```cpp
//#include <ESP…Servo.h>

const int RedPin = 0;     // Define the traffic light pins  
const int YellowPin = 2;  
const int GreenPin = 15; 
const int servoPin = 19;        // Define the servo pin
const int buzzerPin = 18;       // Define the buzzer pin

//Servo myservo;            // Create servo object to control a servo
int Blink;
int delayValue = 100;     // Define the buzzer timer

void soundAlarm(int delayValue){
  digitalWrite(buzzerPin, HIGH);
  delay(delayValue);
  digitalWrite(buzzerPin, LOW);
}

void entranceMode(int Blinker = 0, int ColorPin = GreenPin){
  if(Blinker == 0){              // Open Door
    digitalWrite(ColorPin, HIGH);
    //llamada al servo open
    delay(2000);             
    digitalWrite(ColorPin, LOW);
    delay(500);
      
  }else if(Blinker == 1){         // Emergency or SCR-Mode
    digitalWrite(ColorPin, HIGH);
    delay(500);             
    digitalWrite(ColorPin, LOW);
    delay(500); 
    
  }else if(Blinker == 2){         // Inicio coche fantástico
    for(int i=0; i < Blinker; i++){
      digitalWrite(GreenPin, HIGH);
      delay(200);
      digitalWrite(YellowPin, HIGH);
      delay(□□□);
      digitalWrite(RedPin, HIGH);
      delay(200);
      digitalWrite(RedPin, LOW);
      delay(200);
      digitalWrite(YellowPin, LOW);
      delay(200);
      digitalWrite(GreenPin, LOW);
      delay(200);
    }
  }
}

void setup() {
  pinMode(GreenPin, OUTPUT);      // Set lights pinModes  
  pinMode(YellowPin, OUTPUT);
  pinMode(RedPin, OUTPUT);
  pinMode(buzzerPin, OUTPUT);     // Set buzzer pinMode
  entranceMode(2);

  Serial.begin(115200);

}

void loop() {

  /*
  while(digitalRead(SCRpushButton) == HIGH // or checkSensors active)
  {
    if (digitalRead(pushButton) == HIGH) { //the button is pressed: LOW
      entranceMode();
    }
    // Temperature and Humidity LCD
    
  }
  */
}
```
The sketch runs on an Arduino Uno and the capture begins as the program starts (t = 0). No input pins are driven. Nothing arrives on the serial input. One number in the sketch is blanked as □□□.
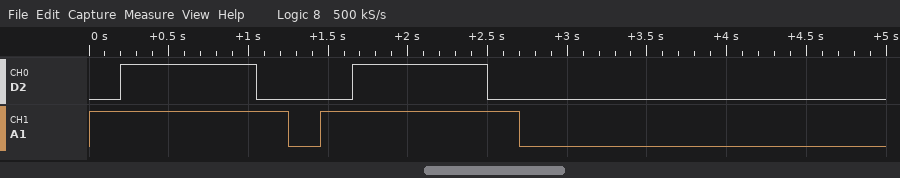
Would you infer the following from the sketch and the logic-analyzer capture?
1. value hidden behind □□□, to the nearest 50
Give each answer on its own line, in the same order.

450
